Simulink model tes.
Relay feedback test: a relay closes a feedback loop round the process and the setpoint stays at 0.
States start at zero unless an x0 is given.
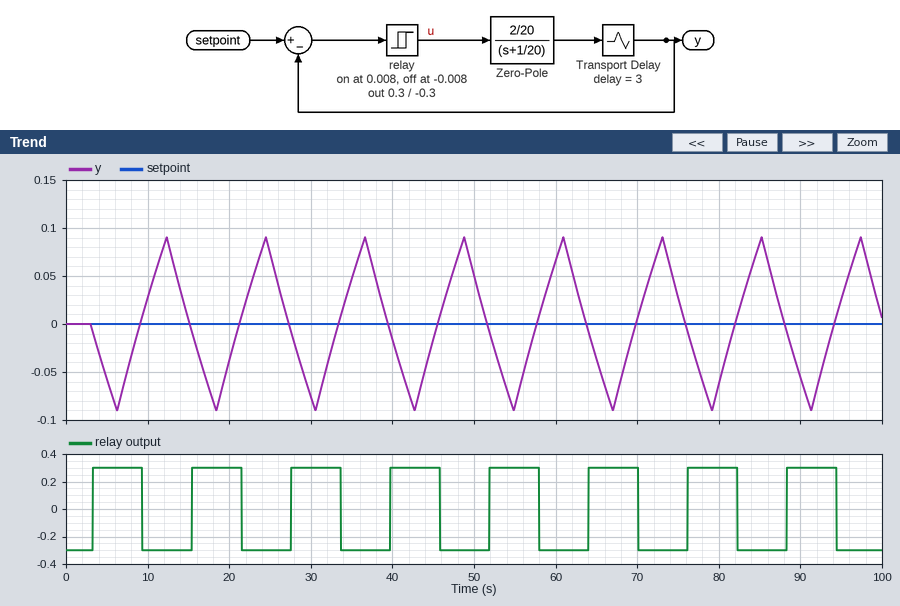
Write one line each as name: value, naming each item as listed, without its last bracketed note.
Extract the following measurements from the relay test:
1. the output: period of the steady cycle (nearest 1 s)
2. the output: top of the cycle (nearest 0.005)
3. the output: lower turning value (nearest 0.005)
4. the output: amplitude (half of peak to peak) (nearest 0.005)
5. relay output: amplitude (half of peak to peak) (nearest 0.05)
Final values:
the output: period of the steady cycle: 12 s
the output: top of the cycle: 0.090
the output: lower turning value: -0.090
the output: amplitude (half of peak to peak): 0.090
relay output: amplitude (half of peak to peak): 0.30
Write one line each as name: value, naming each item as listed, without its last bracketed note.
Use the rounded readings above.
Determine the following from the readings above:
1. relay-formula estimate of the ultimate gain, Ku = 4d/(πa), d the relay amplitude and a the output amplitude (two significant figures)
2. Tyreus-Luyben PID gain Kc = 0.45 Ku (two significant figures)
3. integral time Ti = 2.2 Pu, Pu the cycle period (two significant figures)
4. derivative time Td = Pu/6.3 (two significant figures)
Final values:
relay-formula estimate of the ultimate gain, Ku = 4d/(πa), d the relay amplitude and a the output amplitude: 4.2
Tyreus-Luyben PID gain Kc = 0.45 Ku: 1.9
integral time Ti = 2.2 Pu, Pu the cycle period: 26 s
derivative time Td = Pu/6.3: 1.9 s
